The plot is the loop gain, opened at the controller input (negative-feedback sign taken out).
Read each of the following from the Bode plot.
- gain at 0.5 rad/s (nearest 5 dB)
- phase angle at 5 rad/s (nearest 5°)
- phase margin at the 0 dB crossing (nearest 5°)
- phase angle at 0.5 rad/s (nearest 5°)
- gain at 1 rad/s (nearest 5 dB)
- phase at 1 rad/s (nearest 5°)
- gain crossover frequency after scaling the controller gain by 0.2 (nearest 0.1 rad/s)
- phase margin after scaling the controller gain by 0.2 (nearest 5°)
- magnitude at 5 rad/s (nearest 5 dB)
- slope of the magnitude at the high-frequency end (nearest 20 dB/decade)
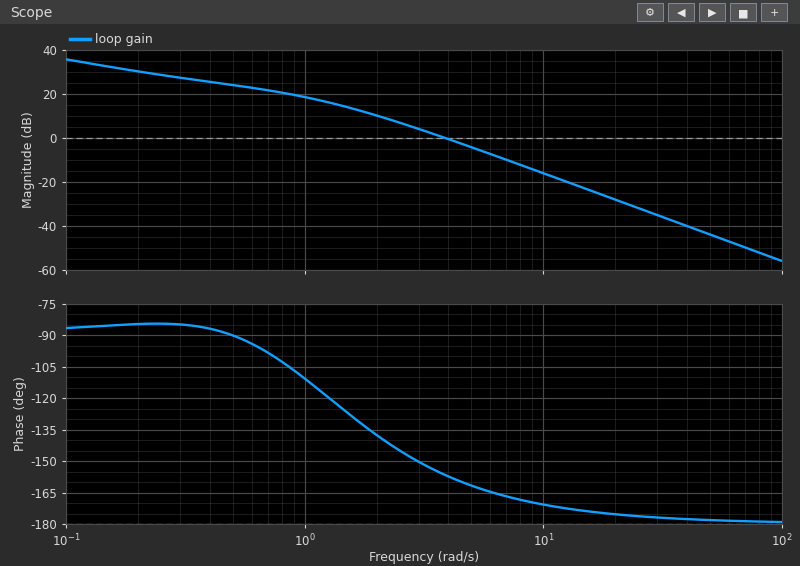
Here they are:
25 dB
-160°
25°
-90°
20 dB
-110°
1.5 rad/s
55°
-5 dB
-40 dB/decade
